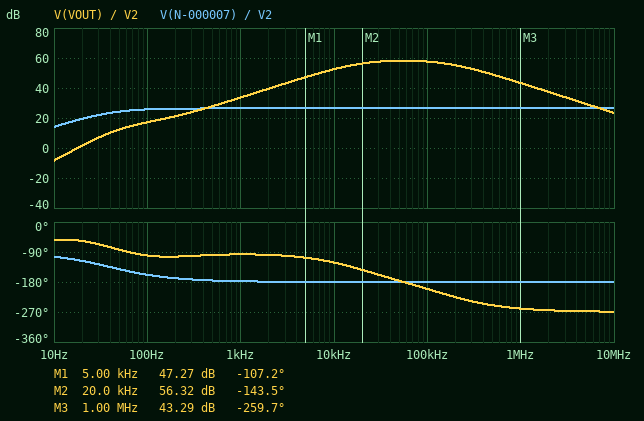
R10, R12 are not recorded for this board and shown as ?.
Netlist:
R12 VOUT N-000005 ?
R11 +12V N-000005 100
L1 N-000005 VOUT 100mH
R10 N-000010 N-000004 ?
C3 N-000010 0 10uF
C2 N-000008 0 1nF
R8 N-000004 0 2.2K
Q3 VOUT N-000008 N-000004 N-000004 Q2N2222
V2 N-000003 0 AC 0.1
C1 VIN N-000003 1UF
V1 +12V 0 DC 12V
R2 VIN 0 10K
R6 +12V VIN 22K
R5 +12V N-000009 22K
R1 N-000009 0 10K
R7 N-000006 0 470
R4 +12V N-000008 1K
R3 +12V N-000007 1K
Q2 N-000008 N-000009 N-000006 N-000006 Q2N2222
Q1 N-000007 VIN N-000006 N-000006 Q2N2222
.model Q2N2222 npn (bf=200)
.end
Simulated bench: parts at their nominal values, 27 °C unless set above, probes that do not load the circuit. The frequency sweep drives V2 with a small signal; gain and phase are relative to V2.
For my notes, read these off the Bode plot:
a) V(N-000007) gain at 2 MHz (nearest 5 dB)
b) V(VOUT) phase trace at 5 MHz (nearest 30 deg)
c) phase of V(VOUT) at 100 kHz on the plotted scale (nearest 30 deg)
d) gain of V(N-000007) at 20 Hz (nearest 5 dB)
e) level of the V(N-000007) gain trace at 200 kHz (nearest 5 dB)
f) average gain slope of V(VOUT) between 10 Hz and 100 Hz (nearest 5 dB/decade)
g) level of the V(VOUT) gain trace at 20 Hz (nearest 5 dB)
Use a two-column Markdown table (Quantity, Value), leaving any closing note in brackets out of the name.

| Quantity | Value |
|---|---|
| V(N-000007) gain at 2 MHz | 25 dB |
| V(VOUT) phase trace at 5 MHz | -270 deg |
| phase of V(VOUT) at 100 kHz on the plotted scale | -210 deg |
| gain of V(N-000007) at 20 Hz | 20 dB |
| level of the V(N-000007) gain trace at 200 kHz | 25 dB |
| average gain slope of V(VOUT) between 10 Hz and 100 Hz | 25 dB/decade |
| level of the V(VOUT) gain trace at 20 Hz | 0 dB |
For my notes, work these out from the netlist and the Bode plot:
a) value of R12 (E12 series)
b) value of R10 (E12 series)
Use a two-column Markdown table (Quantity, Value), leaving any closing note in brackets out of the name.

| Quantity | Value |
|---|---|
| value of R12 | 12 kΩ |
| value of R10 | 270 Ω |
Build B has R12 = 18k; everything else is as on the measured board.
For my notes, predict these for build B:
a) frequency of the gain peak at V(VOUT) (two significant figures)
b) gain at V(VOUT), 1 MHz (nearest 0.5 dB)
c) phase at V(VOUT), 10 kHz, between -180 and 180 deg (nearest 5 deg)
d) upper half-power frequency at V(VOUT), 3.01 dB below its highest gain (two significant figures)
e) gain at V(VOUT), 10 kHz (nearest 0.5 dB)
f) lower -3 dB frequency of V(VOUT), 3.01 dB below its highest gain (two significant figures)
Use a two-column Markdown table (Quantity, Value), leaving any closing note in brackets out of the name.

| Quantity | Value |
|---|---|
| frequency of the gain peak at V(VOUT) | 68 kHz |
| gain at V(VOUT), 1 MHz | 47.0 dB |
| phase at V(VOUT), 10 kHz, between -180 and 180 deg | -115 deg |
| upper half-power frequency at V(VOUT), 3.01 dB below its highest gain | 210 kHz |
| gain at V(VOUT), 10 kHz | 53.0 dB |
| lower -3 dB frequency of V(VOUT), 3.01 dB below its highest gain | 22 kHz |
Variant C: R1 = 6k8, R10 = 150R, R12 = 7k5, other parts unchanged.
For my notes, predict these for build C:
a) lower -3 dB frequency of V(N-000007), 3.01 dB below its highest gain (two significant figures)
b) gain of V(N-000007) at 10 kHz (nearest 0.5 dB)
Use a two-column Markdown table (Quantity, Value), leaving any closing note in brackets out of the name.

| Quantity | Value |
|---|---|
| lower -3 dB frequency of V(N-000007), 3.01 dB below its highest gain | 25 Hz |
| gain of V(N-000007) at 10 kHz | 6.5 dB |
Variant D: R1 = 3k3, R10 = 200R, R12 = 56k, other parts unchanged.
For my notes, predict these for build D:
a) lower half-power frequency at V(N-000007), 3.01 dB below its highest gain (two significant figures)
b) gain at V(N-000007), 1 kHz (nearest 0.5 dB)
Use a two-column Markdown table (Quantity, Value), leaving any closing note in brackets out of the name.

| Quantity | Value |
|---|---|
| lower half-power frequency at V(N-000007), 3.01 dB below its highest gain | 25 Hz |
| gain at V(N-000007), 1 kHz | 6.5 dB |
